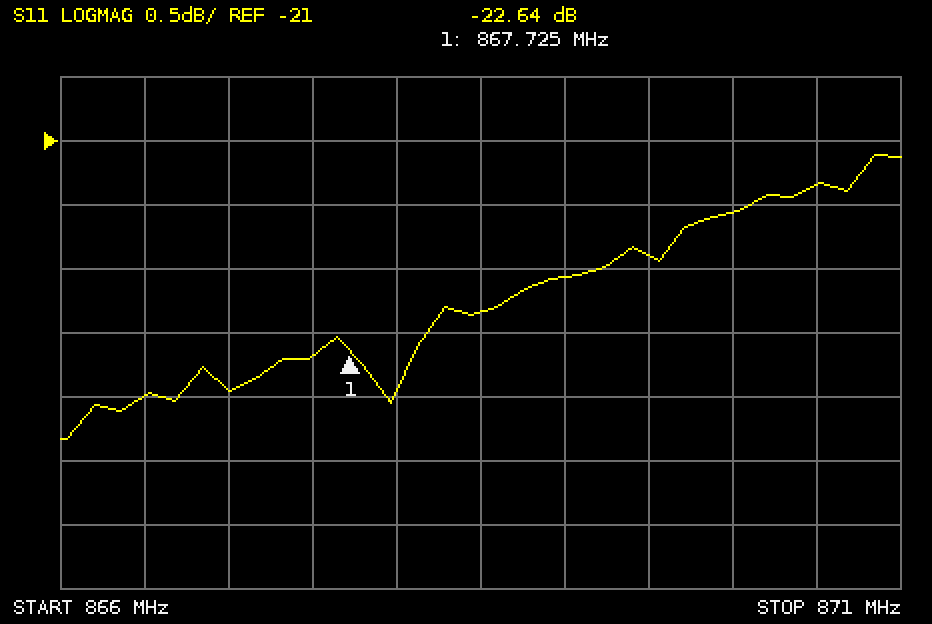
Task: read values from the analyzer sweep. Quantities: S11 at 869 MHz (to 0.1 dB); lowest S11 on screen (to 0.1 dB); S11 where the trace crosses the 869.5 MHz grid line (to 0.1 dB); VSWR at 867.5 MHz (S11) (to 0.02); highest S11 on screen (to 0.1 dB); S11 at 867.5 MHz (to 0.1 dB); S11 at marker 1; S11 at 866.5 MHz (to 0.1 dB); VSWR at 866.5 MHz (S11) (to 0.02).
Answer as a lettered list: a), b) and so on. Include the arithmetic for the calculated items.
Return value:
a) -22.1 dB
b) -23.3 dB
c) -21.9 dB
d) |Γ| = 10^(-22.7/20) = 0.0733; VSWR = (1 + 0.0733)/(1 − 0.0733) ≈ 1.16
e) -21.1 dB
f) -22.7 dB
g) -22.64 dB
h) -23.0 dB
i) |Γ| = 10^(-23/20) = 0.0708; VSWR = (1 + 0.0708)/(1 − 0.0708) ≈ 1.15, so 1.16 to the nearest 0.02
